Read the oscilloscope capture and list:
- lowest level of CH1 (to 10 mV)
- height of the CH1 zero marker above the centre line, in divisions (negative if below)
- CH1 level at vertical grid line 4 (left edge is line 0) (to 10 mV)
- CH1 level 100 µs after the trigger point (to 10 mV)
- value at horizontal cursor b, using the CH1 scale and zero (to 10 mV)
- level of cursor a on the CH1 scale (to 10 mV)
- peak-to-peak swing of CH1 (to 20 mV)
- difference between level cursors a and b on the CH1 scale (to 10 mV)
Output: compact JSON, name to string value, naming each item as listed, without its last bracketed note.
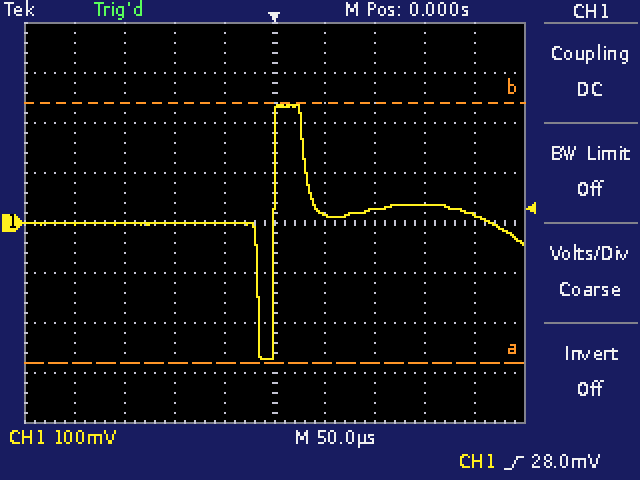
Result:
{"lowest level of CH1": "-270 mV", "height of the CH1 zero marker above the centre line, in divisions": "0.0 div", "CH1 level at vertical grid line 4 (left edge is line 0)": "0 mV", "CH1 level 100 µs after the trigger point": "30 mV", "value at horizontal cursor b, using the CH1 scale and zero": "240 mV", "level of cursor a on the CH1 scale": "-280 mV", "peak-to-peak swing of CH1": "500 mV", "difference between level cursors a and b on the CH1 scale": "520 mV"}
